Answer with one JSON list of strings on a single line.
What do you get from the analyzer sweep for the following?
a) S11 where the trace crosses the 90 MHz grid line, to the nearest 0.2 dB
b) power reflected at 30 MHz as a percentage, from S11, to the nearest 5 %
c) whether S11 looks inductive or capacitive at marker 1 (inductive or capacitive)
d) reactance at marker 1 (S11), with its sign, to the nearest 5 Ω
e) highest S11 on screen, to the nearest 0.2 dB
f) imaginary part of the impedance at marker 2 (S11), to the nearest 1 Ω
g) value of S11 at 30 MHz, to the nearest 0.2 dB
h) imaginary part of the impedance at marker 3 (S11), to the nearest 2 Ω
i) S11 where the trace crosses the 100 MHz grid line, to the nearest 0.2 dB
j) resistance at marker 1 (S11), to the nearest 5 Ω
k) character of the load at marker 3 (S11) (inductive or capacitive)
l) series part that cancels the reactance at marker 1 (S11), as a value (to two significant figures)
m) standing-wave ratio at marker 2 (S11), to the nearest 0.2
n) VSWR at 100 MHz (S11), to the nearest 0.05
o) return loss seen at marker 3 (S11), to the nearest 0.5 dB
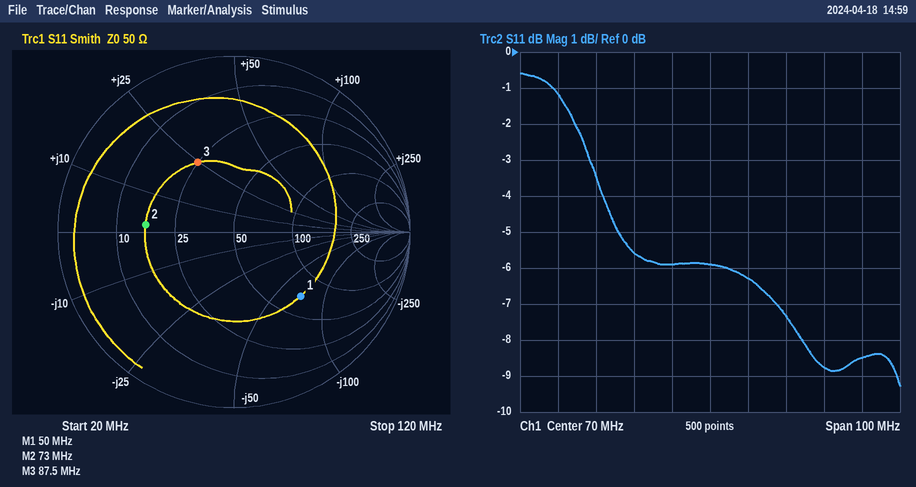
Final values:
["-7.4 dB", "75 %", "capacitive", "-70 Ω", "-0.6 dB", "+2 Ω", "-1.2 dB", "+24 Ω", "-8.8 dB", "70 Ω", "inductive", "220 nH", "3.0", "2.15", "7.0 dB"]
